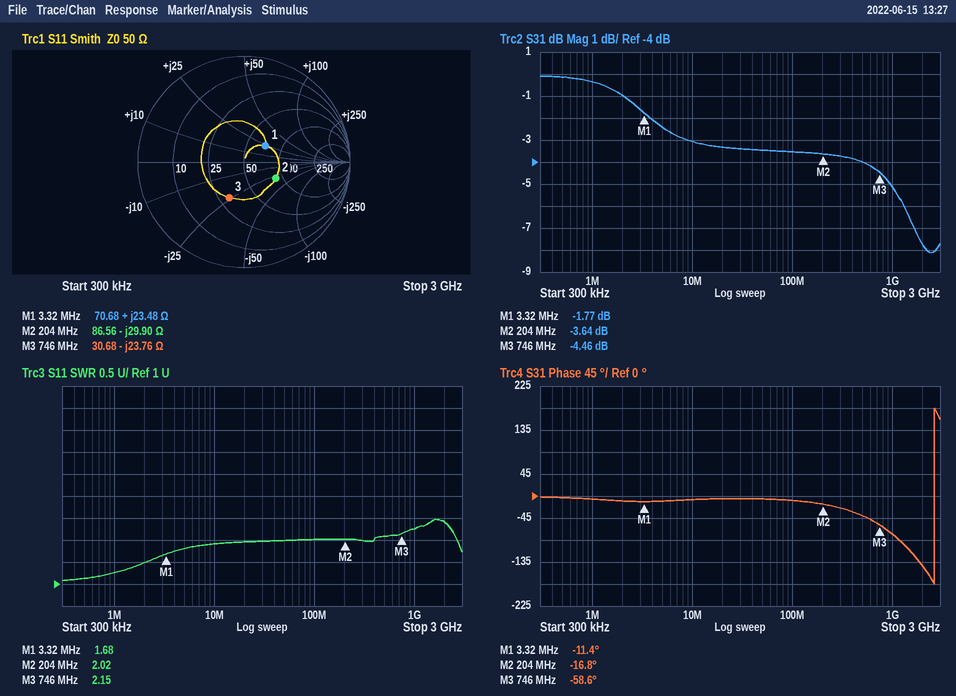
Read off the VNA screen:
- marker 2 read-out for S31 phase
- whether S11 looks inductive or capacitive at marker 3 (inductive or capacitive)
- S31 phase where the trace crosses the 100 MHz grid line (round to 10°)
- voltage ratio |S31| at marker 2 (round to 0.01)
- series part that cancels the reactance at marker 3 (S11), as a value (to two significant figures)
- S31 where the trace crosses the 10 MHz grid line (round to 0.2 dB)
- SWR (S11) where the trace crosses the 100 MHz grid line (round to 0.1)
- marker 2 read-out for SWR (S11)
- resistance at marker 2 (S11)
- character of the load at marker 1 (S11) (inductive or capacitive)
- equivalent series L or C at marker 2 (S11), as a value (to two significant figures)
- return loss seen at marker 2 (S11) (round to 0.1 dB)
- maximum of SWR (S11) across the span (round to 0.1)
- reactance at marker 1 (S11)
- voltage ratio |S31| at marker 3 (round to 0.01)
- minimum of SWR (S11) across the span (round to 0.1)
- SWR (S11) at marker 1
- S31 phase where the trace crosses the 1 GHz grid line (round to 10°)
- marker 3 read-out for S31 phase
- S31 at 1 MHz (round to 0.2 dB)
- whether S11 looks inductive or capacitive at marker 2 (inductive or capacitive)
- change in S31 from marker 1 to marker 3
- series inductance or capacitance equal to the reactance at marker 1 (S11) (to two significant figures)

-16.8°
capacitive
-10°
0.66
5.1 nH
-3.0 dB
2.0
2.02
86.56 Ω
inductive
26 pF
9.4 dB
2.5
+23.48 Ω
0.60
1.1
1.68
-80°
-58.6°
-0.4 dB
capacitive
-2.69 dB
1.1 µH
